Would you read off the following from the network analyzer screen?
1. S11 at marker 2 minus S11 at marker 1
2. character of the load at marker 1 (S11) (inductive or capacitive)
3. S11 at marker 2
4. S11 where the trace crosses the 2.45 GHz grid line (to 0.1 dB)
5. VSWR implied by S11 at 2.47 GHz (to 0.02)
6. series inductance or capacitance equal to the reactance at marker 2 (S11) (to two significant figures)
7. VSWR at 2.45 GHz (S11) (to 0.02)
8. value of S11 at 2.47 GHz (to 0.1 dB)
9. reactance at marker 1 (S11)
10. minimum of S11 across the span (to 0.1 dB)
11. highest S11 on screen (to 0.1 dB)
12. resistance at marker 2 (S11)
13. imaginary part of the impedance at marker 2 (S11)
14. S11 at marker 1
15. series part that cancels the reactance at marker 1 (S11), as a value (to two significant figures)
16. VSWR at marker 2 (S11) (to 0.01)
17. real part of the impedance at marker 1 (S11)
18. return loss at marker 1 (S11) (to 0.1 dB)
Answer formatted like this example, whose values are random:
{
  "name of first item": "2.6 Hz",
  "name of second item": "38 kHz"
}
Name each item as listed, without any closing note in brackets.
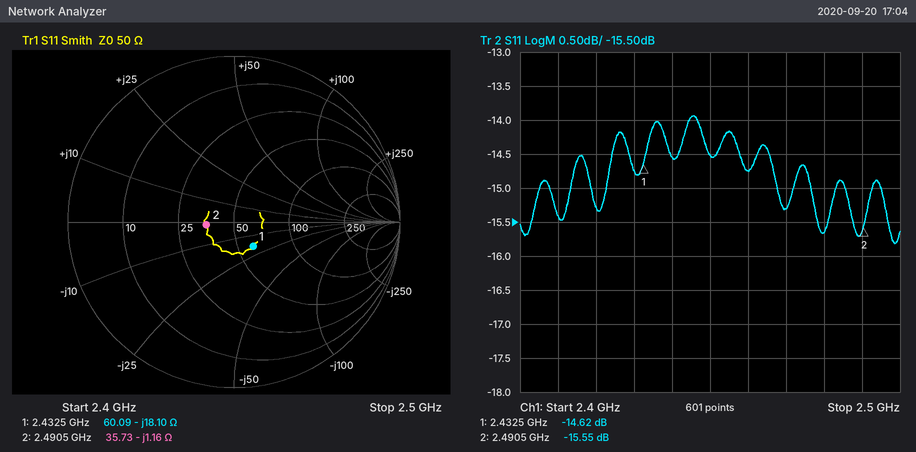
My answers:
{
  "S11 at marker 2 minus S11 at marker 1": "-0.93 dB",
  "character of the load at marker 1 (S11)": "capacitive",
  "S11 at marker 2": "-15.55 dB",
  "S11 where the trace crosses the 2.45 GHz grid line": "-14.5 dB",
  "VSWR implied by S11 at 2.47 GHz": "1.42",
  "series inductance or capacitance equal to the reactance at marker 2 (S11)": "55 pF",
  "VSWR at 2.45 GHz (S11)": "1.46",
  "value of S11 at 2.47 GHz": "-15.3 dB",
  "reactance at marker 1": "-18.10 Ω",
  "minimum of S11 across the span": "-15.8 dB",
  "highest S11 on screen": "-13.9 dB",
  "resistance at marker 2": "35.73 Ω",
  "imaginary part of the impedance at marker 2": "-1.16 Ω",
  "S11 at marker 1": "-14.62 dB",
  "series part that cancels the reactance at marker 1 (S11), as a value": "1.2 nH",
  "VSWR at marker 2 (S11)": "1.40",
  "real part of the impedance at marker 1": "60.09 Ω",
  "return loss at marker 1 (S11)": "14.6 dB"
}
